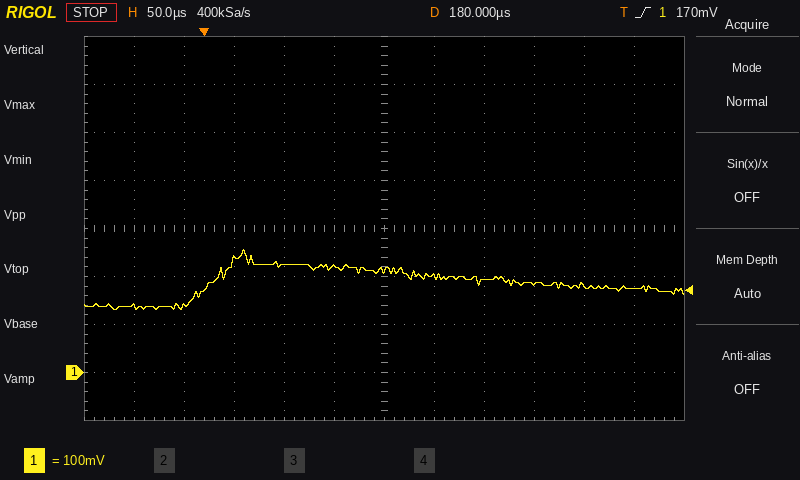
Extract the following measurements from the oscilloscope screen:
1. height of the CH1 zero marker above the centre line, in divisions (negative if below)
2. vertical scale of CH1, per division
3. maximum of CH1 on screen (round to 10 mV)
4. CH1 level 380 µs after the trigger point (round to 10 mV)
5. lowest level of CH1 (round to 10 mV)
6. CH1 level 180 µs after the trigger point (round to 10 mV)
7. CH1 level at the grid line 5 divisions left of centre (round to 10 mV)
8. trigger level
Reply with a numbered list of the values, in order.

1. -3.0 div
2. 100 mV
3. 260 mV
4. 180 mV
5. 130 mV
6. 210 mV
7. 140 mV
8. 170 mV
